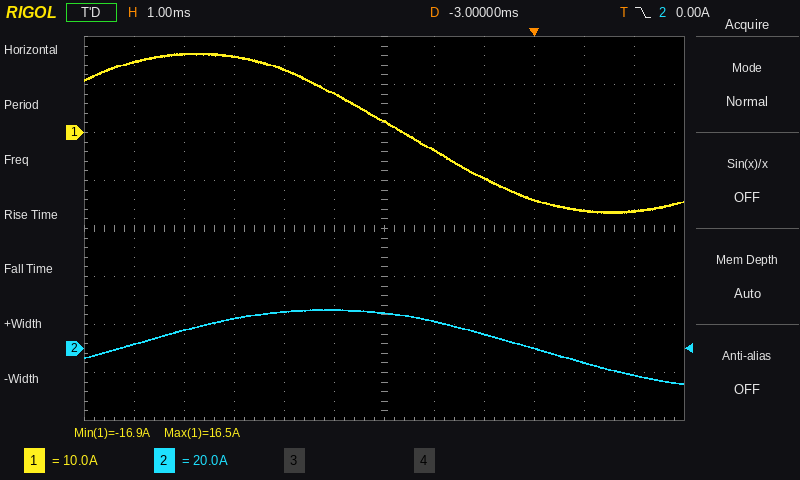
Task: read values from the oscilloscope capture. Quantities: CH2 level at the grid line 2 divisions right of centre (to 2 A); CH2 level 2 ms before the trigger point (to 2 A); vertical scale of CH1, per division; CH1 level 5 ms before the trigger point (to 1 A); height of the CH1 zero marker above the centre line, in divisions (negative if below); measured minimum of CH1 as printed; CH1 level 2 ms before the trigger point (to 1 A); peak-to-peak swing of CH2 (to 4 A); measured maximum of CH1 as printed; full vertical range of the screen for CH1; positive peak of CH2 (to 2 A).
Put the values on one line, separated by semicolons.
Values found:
6 A; 12 A; 10 A; 13 A; +2.0 div; -16.9 A; -4 A; 32 A; 16.5 A; 80 A; 16 A
